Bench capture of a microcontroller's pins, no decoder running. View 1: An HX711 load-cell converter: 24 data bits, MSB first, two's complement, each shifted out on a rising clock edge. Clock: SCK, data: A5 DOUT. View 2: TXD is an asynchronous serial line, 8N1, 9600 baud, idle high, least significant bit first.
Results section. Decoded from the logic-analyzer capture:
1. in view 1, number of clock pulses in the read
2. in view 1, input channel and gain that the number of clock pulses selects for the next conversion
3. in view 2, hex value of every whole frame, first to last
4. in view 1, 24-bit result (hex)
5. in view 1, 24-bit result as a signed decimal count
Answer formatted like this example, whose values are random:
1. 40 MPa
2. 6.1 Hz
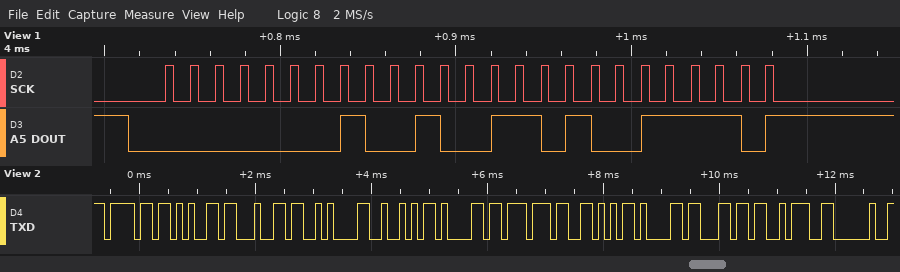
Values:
1. 25
2. channel A, gain 128
3. 6F 65 64 0A 52 61 77 56 61 6C 3A 20
4. 0x01269E
5. 75422
